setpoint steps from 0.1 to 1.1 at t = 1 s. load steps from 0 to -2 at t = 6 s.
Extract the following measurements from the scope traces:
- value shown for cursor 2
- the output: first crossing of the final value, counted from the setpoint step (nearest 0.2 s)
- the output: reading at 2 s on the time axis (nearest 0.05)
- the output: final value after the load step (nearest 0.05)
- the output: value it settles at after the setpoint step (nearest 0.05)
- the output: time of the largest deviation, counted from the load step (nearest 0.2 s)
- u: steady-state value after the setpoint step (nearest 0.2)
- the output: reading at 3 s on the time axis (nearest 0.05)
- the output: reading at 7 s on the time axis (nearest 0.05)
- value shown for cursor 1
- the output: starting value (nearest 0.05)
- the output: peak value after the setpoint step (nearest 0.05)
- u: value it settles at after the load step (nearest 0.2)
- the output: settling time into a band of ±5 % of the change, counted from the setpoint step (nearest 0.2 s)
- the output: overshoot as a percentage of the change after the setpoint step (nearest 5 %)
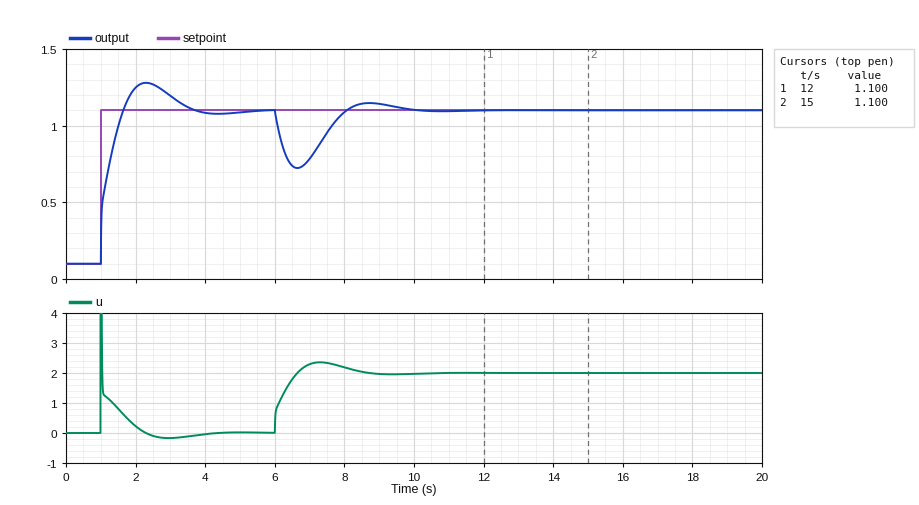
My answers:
1.100
0.6 s
1.25
1.10
1.10
0.6 s
0.0
1.20
0.80
1.100
0.10
1.30
2.0
2.2 s
20 %
